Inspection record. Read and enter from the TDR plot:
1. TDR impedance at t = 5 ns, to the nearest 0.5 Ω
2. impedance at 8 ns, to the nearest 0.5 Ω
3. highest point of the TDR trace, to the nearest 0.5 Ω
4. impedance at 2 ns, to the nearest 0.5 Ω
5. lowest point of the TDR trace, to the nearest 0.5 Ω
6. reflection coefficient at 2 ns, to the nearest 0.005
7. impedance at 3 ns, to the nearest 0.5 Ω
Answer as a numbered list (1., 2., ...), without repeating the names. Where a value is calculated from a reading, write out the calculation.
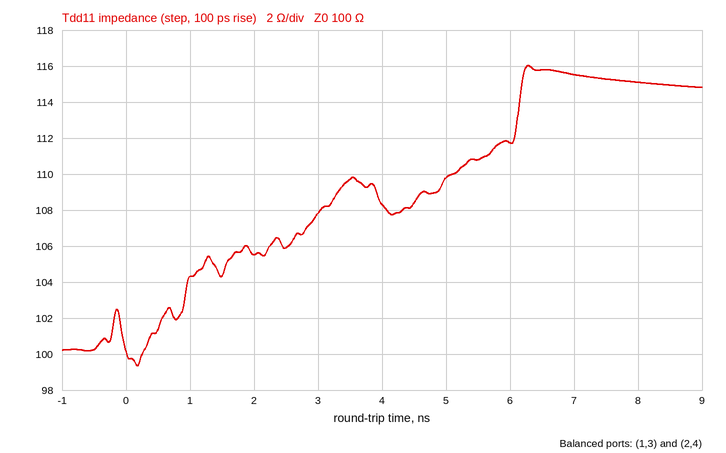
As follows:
1. 110.0 Ω
2. 115.0 Ω
3. 116.0 Ω
4. 105.5 Ω
5. 99.5 Ω
6. (105.5 − 100)/(105.5 + 100) ≈ +0.0268, so +0.025 to the nearest 0.005
7. 108.0 Ω
